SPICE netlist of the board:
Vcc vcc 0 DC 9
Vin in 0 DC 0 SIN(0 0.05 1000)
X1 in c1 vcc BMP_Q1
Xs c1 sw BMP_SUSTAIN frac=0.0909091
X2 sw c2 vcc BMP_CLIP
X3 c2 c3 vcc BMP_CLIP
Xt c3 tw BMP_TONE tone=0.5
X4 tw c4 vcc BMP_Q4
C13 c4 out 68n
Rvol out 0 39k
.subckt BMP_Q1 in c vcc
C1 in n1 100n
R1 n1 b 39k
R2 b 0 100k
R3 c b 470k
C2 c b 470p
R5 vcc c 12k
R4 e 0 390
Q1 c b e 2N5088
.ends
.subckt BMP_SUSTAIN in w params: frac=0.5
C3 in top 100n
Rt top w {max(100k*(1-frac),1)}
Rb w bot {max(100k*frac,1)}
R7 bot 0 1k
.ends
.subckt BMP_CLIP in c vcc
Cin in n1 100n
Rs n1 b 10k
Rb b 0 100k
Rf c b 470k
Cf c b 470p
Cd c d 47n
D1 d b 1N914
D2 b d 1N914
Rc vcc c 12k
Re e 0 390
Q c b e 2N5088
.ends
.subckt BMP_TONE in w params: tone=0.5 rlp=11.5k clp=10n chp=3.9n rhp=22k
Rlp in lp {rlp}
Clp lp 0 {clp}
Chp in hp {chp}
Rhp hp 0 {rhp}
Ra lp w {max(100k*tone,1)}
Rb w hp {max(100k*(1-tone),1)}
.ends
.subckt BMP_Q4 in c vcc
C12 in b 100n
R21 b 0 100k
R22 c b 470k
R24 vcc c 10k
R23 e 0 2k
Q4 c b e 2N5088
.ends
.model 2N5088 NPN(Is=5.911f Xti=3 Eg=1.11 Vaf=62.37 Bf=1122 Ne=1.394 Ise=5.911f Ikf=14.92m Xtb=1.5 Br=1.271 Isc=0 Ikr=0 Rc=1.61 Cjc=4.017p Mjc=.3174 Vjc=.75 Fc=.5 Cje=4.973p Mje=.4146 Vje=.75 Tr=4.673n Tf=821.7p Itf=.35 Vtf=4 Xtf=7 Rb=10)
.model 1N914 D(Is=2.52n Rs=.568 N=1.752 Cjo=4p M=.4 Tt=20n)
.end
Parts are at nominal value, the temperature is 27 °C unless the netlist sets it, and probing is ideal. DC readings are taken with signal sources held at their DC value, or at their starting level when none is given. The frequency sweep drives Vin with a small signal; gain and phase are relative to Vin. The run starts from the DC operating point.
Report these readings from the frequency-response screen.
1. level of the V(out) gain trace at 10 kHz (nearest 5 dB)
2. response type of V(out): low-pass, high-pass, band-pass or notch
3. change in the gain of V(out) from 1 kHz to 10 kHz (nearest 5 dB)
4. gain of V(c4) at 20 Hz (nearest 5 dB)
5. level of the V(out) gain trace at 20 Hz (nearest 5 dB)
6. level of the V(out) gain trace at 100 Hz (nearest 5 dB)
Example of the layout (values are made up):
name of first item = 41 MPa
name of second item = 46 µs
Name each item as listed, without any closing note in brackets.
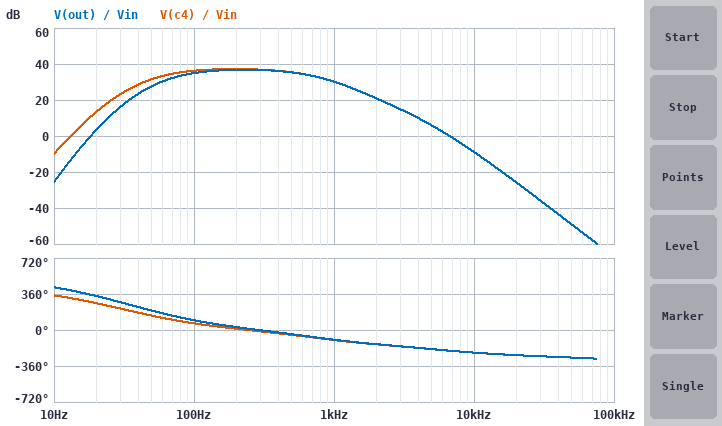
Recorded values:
level of the V(out) gain trace at 10 kHz = -10 dB
response type of V(out): low-pass, high-pass, band-pass or notch = band-pass
change in the gain of V(out) from 1 kHz to 10 kHz = -40 dB
gain of V(c4) at 20 Hz = 15 dB
level of the V(out) gain trace at 20 Hz = 5 dB
level of the V(out) gain trace at 100 Hz = 35 dB
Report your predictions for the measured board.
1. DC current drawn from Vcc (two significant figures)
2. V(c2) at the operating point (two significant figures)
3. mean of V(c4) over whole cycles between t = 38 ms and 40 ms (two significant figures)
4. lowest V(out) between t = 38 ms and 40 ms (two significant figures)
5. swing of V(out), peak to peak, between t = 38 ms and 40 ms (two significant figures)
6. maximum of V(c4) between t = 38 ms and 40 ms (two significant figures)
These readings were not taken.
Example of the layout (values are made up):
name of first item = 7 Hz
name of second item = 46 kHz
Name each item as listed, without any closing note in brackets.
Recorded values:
DC current drawn from Vcc = 1.3 mA
V(c2) at the operating point = 4.7 V
mean of V(c4) over whole cycles between t = 38 ms and 40 ms = 6.5 V
lowest V(out) between t = 38 ms and 40 ms = -380 mV
swing of V(out), peak to peak, between t = 38 ms and 40 ms = 760 mV
maximum of V(c4) between t = 38 ms and 40 ms = 6.9 V
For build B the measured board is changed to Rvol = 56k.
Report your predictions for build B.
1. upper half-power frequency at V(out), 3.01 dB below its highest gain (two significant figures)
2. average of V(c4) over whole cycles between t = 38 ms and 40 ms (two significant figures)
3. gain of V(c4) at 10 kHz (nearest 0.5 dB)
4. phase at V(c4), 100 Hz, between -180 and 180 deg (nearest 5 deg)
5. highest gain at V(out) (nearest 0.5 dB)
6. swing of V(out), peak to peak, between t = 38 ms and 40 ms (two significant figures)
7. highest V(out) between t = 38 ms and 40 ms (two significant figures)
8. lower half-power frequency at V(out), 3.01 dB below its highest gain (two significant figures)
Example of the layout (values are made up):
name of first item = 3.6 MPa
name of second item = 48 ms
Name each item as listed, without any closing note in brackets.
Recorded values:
upper half-power frequency at V(out), 3.01 dB below its highest gain = 650 Hz
average of V(c4) over whole cycles between t = 38 ms and 40 ms = 6.5 V
gain of V(c4) at 10 kHz = -8.5 dB
phase at V(c4), 100 Hz, between -180 and 180 deg = 70 deg
highest gain at V(out) = 37.5 dB
swing of V(out), peak to peak, between t = 38 ms and 40 ms = 810 mV
highest V(out) between t = 38 ms and 40 ms = 400 mV
lower half-power frequency at V(out), 3.01 dB below its highest gain = 79 Hz
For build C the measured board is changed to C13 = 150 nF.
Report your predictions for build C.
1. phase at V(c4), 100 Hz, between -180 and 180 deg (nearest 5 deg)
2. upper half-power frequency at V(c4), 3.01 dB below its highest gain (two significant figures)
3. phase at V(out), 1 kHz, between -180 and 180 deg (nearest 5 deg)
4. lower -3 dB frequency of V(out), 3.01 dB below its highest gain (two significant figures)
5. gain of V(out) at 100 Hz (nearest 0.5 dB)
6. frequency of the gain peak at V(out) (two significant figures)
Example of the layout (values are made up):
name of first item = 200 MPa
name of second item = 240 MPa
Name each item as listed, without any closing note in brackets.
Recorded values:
phase at V(c4), 100 Hz, between -180 and 180 deg = 70 deg
upper half-power frequency at V(c4), 3.01 dB below its highest gain = 640 Hz
phase at V(out), 1 kHz, between -180 and 180 deg = -100 deg
lower -3 dB frequency of V(out), 3.01 dB below its highest gain = 75 Hz
gain of V(out) at 100 Hz = 35.5 dB
frequency of the gain peak at V(out) = 210 Hz
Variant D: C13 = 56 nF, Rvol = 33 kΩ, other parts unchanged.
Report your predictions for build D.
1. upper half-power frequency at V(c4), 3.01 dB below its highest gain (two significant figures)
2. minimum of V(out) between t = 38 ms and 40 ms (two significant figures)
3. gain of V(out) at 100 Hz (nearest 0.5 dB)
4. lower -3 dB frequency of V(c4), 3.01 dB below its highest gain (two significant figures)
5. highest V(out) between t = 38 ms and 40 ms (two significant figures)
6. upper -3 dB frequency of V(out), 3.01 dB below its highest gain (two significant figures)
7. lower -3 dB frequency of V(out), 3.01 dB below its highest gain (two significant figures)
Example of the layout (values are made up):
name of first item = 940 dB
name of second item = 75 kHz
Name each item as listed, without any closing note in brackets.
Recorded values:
upper half-power frequency at V(c4), 3.01 dB below its highest gain = 610 Hz
minimum of V(out) between t = 38 ms and 40 ms = -370 mV
gain of V(out) at 100 Hz = 34.0 dB
lower -3 dB frequency of V(c4), 3.01 dB below its highest gain = 64 Hz
highest V(out) between t = 38 ms and 40 ms = 370 mV
upper -3 dB frequency of V(out), 3.01 dB below its highest gain = 670 Hz
lower -3 dB frequency of V(out), 3.01 dB below its highest gain = 93 Hz
